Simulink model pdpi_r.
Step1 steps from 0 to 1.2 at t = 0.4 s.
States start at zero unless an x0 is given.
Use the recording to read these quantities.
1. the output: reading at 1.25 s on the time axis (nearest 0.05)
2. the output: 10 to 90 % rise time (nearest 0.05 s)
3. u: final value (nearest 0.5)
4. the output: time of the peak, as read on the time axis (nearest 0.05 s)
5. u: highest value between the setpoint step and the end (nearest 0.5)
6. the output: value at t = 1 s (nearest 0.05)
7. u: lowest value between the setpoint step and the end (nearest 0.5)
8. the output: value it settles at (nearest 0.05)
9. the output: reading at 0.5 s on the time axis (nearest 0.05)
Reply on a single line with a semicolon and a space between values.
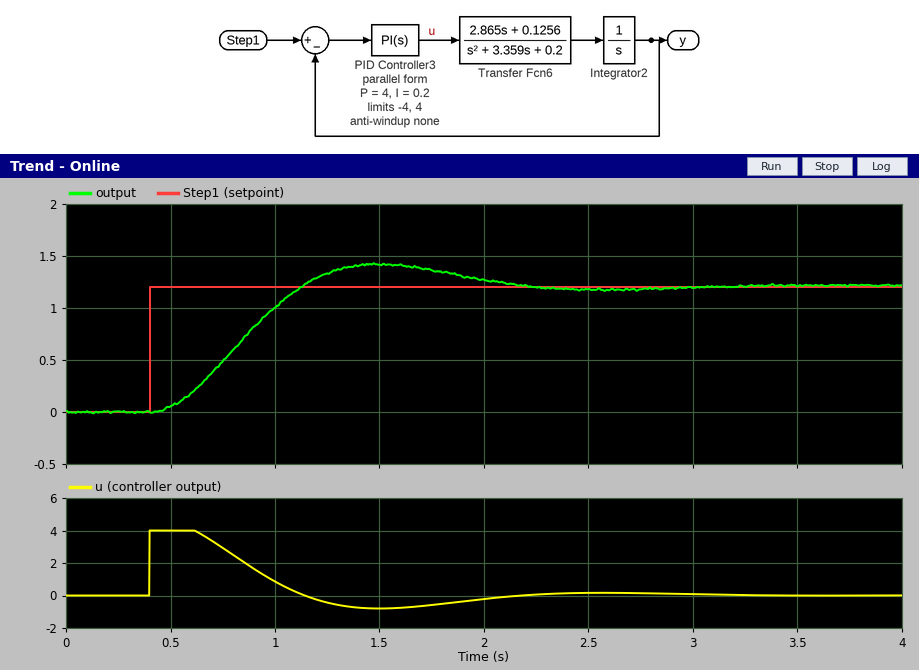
1.35; 0.50 s; 0.0; 1.50 s; 4.0; 1.00; -1.0; 1.20; 0.05
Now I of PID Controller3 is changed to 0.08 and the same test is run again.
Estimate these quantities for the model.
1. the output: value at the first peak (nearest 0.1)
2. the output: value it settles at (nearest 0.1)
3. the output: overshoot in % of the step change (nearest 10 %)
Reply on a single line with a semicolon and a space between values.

1.4; 1.2; 20 %
